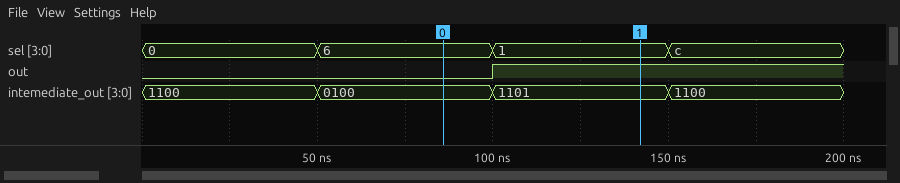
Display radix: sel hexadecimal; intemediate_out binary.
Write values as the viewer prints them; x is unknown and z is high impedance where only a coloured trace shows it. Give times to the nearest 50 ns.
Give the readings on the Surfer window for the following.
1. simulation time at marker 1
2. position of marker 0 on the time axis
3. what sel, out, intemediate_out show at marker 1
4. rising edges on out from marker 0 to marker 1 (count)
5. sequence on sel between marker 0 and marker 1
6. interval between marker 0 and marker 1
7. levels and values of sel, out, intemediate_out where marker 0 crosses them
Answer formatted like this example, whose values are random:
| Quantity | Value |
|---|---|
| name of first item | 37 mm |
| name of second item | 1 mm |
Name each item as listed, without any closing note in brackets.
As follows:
| Quantity | Value |
|---|---|
| simulation time at marker 1 | 150 ns |
| position of marker 0 on the time axis | 100 ns |
| what sel, out, intemediate_out show at marker 1 | sel=1, out=1, intemediate_out=1101 |
| rising edges on out from marker 0 to marker 1 | 1 |
| sequence on sel between marker 0 and marker 1 | 6, 1 |
| interval between marker 0 and marker 1 | 50 ns |
| levels and values of sel, out, intemediate_out where marker 0 crosses them | sel=6, out=0, intemediate_out=0100 |
